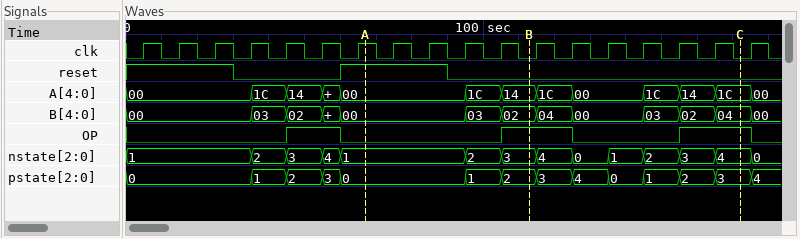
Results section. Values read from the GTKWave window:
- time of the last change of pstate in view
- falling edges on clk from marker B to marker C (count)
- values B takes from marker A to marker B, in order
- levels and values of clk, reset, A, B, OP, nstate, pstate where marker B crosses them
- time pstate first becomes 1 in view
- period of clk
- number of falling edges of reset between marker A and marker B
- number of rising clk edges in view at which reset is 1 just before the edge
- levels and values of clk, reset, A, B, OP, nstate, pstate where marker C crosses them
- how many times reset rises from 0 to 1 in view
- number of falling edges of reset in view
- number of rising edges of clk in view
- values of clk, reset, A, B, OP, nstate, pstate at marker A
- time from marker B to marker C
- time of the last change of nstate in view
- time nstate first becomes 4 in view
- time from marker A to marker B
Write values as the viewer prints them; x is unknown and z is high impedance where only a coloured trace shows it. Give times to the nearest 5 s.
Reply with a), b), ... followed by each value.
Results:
a) 175 s
b) 6
c) 00, 03, 02
d) clk=0, reset=0, A=14, B=02, OP=1, nstate=3, pstate=2
e) 35 s
f) 10 s
g) 1
h) 6
i) clk=0, reset=0, A=1C, B=04, OP=1, nstate=4, pstate=3
j) 1
k) 2
l) 18
m) clk=1, reset=1, A=00, B=00, OP=0, nstate=1, pstate=0
n) 60 s
o) 175 s
p) 55 s
q) 45 s
